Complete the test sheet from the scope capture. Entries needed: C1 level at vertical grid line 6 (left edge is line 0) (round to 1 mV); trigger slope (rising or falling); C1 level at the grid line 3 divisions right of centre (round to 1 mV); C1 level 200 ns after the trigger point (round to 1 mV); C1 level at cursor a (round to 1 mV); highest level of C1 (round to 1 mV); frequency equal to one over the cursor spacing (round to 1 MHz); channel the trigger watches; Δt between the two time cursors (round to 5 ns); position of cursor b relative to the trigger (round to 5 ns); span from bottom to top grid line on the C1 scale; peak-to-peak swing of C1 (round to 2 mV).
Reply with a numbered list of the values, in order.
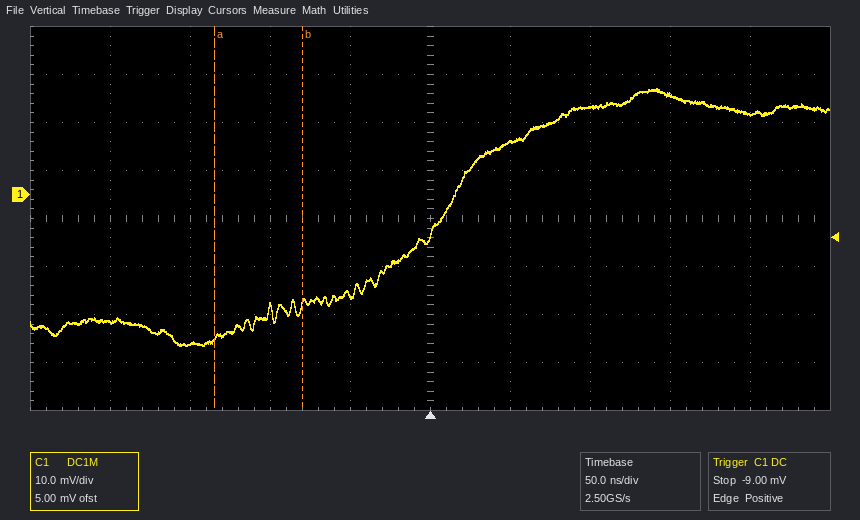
1. 11 mV
2. rising
3. 21 mV
4. 17 mV
5. -30 mV
6. 22 mV
7. 18 MHz
8. C1
9. 55 ns
10. -80 ns
11. 80 mV
12. 54 mV
